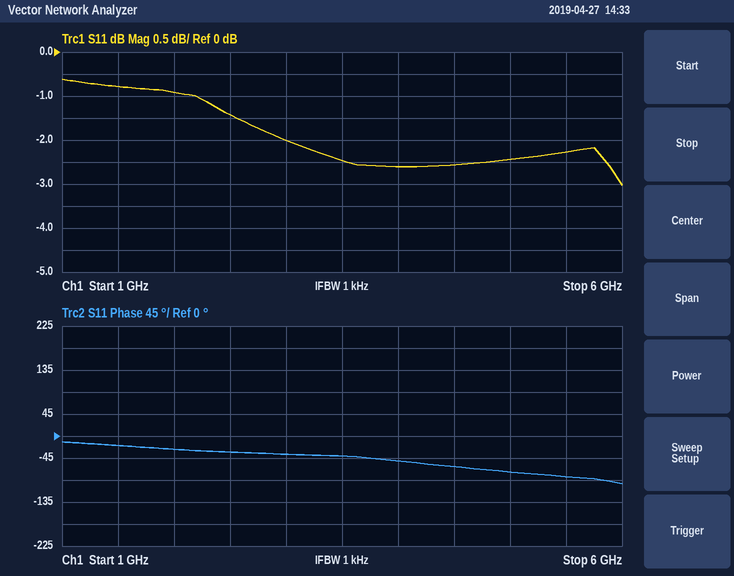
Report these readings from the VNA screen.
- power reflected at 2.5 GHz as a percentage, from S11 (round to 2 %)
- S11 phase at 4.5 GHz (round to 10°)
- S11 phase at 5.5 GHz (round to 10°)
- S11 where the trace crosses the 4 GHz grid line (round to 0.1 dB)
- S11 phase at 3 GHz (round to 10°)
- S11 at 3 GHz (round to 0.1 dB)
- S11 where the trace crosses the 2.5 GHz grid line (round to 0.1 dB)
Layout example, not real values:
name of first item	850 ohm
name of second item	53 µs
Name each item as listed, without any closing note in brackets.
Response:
power reflected at 2.5 GHz as a percentage, from S11	72 %
S11 phase at 4.5 GHz	-60°
S11 phase at 5.5 GHz	-80°
S11 where the trace crosses the 4 GHz grid line	-2.6 dB
S11 phase at 3 GHz	-40°
S11 at 3 GHz	-2.0 dB
S11 where the trace crosses the 2.5 GHz grid line	-1.4 dB
